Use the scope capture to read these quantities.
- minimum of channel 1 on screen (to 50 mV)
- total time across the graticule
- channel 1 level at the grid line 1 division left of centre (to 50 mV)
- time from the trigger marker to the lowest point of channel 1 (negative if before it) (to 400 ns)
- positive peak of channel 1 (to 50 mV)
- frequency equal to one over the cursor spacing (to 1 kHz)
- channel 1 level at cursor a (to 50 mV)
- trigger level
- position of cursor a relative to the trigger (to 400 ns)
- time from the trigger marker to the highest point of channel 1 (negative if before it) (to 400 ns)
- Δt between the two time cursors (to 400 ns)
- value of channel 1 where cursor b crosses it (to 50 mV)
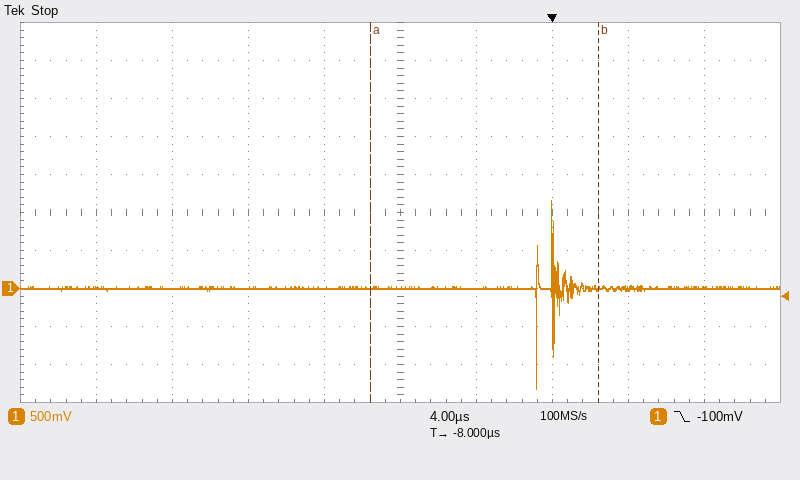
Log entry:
-1.30 V
40 µs
0 mV
-800 ns
1.15 V
83 kHz
0 mV
-100 mV
-9.6 µs
0.0 µs
12.0 µs
0 mV
